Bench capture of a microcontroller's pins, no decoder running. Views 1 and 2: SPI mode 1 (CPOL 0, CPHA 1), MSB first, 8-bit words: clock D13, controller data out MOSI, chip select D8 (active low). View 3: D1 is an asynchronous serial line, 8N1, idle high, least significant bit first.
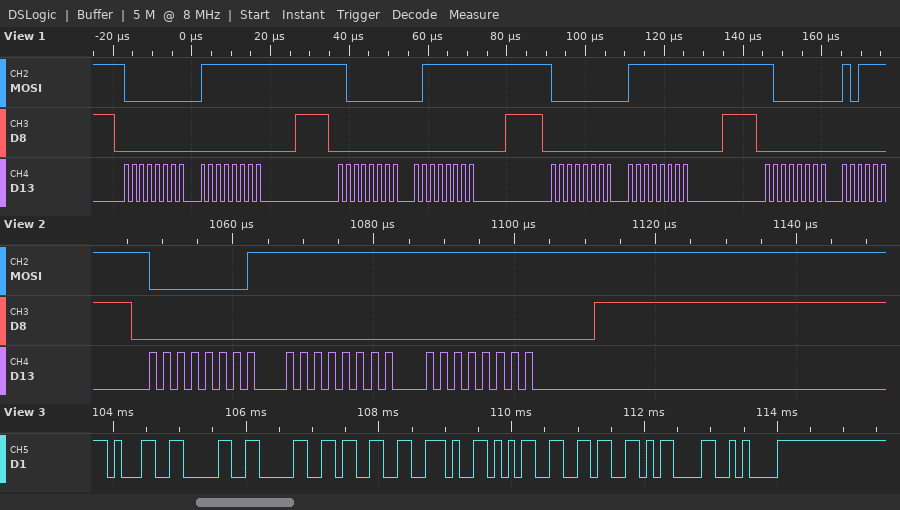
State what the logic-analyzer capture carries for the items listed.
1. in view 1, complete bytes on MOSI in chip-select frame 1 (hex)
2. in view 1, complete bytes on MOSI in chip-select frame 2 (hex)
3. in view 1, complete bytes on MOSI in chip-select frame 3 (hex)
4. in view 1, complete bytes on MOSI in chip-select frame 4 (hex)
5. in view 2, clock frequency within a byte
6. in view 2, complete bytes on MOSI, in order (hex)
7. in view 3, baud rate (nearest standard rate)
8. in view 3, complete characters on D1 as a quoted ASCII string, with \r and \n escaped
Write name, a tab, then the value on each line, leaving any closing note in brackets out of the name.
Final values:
in view 1, complete bytes on MOSI in chip-select frame 1	00 FF
in view 1, complete bytes on MOSI in chip-select frame 2	80 7F
in view 1, complete bytes on MOSI in chip-select frame 3	00 FF
in view 1, complete bytes on MOSI in chip-select frame 4	80
in view 2, clock frequency within a byte	500 kHz
in view 2, complete bytes on MOSI, in order	01 FF FF
in view 3, baud rate	9600 baud
in view 3, complete characters on D1 as a quoted ASCII string, with \r and \n escaped	"1003.56\r\n"
